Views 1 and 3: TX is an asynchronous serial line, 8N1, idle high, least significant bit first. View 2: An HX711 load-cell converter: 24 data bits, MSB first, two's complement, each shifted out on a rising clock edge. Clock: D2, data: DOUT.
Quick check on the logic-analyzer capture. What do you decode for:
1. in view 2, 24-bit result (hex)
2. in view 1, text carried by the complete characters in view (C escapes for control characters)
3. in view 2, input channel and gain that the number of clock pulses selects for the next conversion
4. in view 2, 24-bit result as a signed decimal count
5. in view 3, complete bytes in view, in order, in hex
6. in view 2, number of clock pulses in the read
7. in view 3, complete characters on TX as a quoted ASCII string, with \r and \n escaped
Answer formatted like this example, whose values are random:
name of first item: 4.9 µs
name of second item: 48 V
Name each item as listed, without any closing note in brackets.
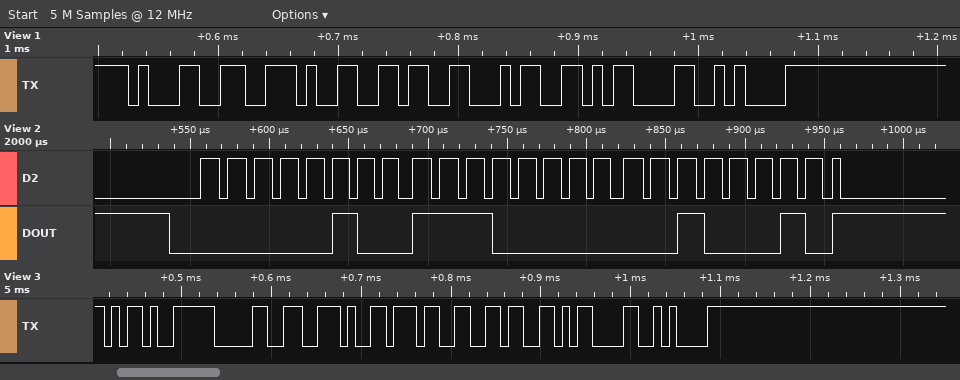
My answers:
in view 2, 24-bit result: 0x04E022
in view 1, text carried by the complete characters in view: "1.64\r\n"
in view 2, input channel and gain that the number of clock pulses selects for the next conversion: channel A, gain 128
in view 2, 24-bit result as a signed decimal count: 319522
in view 3, complete bytes in view, in order, in hex: 2D 30 2E 37 36 0D 0A
in view 2, number of clock pulses in the read: 25
in view 3, complete characters on TX as a quoted ASCII string, with \r and \n escaped: "-0.76\r\n"
